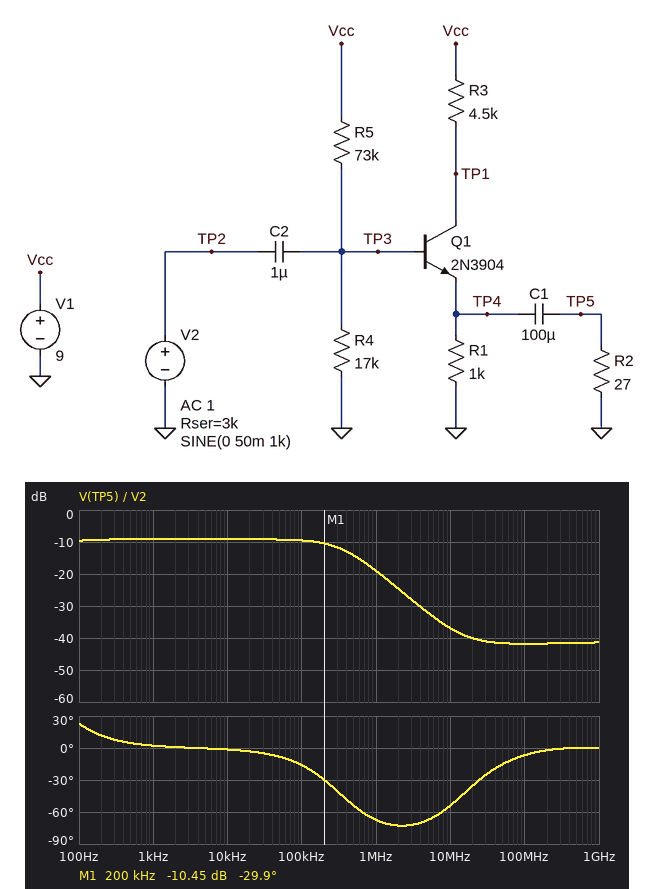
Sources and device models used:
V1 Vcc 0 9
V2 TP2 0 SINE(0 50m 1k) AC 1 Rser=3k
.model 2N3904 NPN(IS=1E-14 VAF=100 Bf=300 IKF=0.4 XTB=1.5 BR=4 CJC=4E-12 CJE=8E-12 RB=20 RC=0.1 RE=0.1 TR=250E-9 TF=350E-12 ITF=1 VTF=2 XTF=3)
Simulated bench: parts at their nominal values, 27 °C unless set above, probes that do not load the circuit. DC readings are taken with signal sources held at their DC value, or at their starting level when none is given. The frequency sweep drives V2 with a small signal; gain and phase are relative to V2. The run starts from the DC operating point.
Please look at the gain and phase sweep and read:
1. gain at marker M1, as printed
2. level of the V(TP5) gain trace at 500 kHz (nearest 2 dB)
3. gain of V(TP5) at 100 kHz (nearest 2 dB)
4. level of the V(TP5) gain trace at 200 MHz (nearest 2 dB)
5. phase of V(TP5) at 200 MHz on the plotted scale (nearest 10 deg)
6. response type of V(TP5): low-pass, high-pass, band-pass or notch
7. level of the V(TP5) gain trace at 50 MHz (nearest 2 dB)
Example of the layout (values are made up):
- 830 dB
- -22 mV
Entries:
- -10.45 dB
- -14 dB
- -10 dB
- -42 dB
- 0 deg
- low-pass
- -42 dB
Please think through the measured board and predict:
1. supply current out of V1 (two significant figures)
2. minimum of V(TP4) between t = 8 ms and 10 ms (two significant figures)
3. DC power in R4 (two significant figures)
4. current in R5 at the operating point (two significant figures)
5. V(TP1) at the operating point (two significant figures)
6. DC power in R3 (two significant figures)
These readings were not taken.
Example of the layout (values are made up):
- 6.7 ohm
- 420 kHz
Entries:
- 1.1 mA
- 990 mV
- 160 µW
- 100 µA
- 4.5 V
- 4.5 mW
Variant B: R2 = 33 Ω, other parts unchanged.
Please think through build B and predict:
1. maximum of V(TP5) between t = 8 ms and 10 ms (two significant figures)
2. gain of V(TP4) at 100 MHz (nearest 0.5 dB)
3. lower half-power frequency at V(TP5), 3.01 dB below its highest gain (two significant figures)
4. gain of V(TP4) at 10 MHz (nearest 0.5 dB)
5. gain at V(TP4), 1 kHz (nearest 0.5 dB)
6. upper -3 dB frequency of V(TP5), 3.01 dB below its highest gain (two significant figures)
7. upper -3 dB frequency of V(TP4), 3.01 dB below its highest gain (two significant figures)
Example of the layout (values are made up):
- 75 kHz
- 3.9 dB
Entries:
- 20 mV
- -40.0 dB
- 33 Hz
- -35.5 dB
- -8.0 dB
- 370 kHz
- 140 kHz
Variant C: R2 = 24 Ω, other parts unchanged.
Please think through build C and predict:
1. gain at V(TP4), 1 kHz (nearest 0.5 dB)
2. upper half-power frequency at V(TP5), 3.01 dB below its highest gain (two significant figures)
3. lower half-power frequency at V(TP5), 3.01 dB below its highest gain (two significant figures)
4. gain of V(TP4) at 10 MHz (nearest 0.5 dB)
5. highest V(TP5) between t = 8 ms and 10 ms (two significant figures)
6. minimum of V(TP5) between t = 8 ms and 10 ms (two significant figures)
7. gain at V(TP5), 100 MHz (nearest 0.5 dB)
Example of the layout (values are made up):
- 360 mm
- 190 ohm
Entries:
- -9.5 dB
- 320 kHz
- 37 Hz
- -38.0 dB
- 17 mV
- -14 mV
- -43.0 dB
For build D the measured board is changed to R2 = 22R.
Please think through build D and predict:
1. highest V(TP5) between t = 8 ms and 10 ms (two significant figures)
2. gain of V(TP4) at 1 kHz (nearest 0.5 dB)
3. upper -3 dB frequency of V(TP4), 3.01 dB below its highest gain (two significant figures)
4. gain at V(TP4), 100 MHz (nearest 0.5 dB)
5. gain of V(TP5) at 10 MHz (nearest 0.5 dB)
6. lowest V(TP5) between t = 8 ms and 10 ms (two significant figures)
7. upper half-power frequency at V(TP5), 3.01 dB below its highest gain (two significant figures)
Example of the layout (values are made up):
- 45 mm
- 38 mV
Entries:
- 16 mV
- -10.0 dB
- 87 Hz
- -43.5 dB
- -38.5 dB
- -13 mV
- 310 kHz
